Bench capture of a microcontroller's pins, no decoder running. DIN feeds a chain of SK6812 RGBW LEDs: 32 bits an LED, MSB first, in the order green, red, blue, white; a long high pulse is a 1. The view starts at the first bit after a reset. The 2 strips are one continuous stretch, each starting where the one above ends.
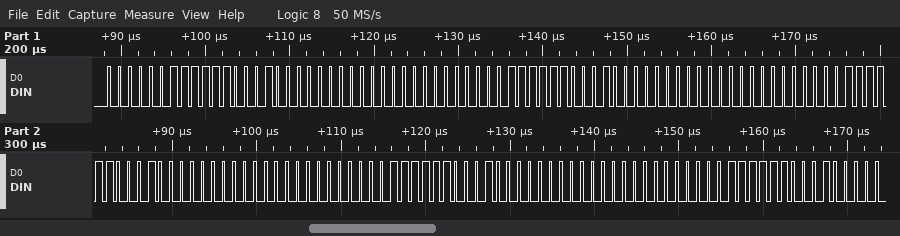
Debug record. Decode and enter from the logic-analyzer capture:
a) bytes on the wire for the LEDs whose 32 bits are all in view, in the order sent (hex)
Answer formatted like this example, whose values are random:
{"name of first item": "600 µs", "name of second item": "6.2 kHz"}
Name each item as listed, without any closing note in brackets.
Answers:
{"bytes on the wire for the LEDs whose 32 bits are all in view, in the order sent": "03 F1 00 00 03 F1 00 00 03 F1 00 00 03 F1 00 00"}
